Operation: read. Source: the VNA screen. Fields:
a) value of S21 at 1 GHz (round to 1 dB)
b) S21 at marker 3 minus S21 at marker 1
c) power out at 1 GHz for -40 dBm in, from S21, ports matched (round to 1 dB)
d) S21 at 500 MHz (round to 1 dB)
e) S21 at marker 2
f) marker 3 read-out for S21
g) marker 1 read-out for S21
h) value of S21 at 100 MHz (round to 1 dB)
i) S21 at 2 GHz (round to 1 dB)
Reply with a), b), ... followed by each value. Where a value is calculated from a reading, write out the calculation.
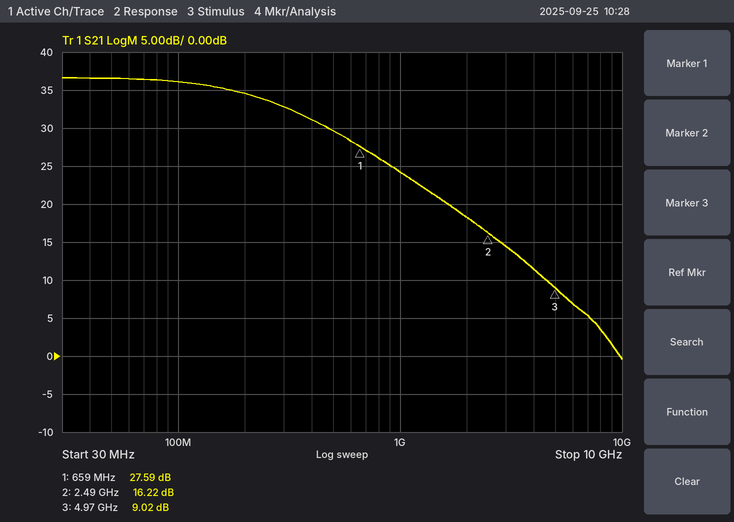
a) 24 dB
b) 9.02 − (27.59) = -18.57 dB
c) -40 dBm + (24 dB) = -16 dBm
d) 30 dB
e) 16.22 dB
f) 9.02 dB
g) 27.59 dB
h) 36 dB
i) 18 dB
